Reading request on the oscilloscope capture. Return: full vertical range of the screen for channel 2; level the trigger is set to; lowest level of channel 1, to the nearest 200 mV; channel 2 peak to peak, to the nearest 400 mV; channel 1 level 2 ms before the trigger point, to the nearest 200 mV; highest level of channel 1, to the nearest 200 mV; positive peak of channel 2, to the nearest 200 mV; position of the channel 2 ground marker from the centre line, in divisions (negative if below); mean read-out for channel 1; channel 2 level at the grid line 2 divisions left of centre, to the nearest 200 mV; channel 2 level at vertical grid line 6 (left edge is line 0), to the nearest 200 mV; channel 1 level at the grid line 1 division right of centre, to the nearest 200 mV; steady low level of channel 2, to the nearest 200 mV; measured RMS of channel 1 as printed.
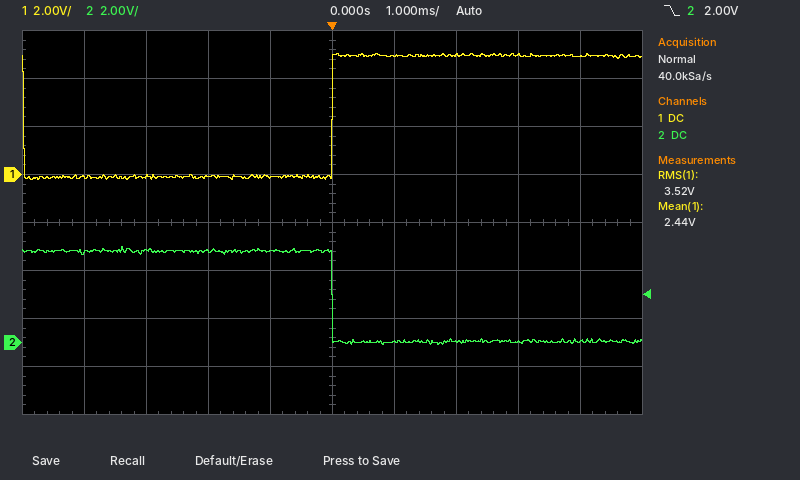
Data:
16 V
2.00 V
-200 mV
4.0 V
0.0 V
5.0 V
4.0 V
-2.5 div
2.44 V
3.8 V
0.0 V
5.0 V
0.0 V
3.52 V
